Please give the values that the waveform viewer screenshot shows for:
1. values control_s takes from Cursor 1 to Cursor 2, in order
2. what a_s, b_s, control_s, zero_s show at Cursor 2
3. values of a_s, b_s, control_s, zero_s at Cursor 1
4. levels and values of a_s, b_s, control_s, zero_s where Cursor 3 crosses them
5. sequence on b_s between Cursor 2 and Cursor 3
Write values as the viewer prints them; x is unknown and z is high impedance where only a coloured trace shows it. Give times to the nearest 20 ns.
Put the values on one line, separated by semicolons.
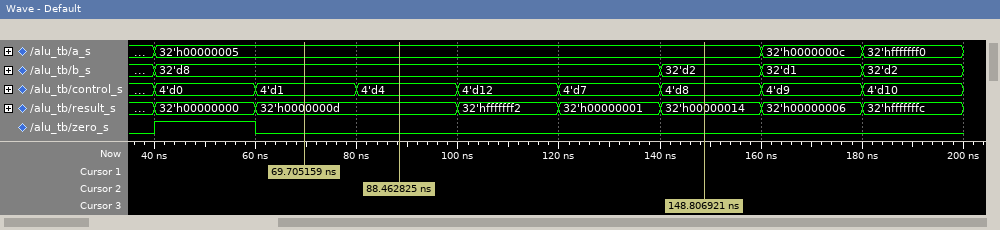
4'd1, 4'd4; a_s=32'h00000005, b_s=32'd8, control_s=4'd4, zero_s=0; a_s=32'h00000005, b_s=32'd8, control_s=4'd1, zero_s=0; a_s=32'h00000005, b_s=32'd2, control_s=4'd8, zero_s=0; 32'd8, 32'd2
